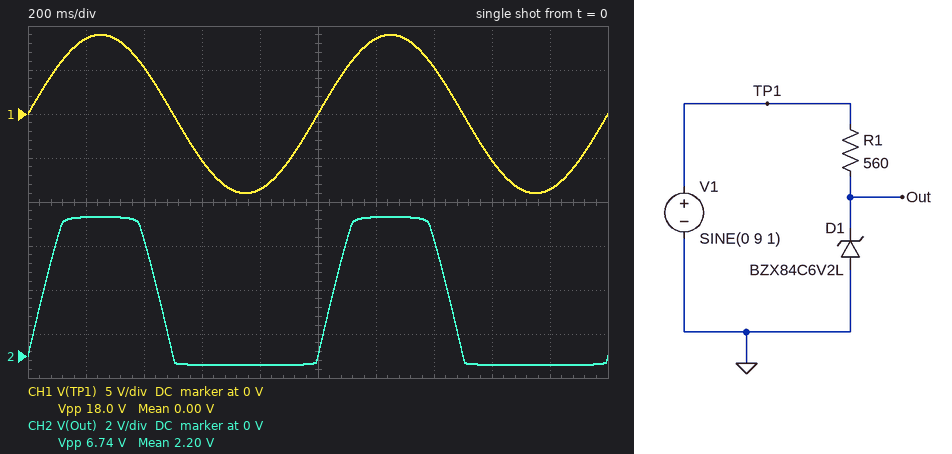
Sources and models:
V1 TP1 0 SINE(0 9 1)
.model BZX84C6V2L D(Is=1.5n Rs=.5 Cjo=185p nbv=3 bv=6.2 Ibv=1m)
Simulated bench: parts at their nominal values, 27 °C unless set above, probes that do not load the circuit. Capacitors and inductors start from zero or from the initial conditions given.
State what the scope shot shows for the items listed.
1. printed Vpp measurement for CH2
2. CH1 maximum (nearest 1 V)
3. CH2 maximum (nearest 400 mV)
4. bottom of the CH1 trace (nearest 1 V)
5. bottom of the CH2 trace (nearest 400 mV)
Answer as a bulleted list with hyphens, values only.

- 6.74 V
- 9 V
- 6.4 V
- -9 V
- -400 mV
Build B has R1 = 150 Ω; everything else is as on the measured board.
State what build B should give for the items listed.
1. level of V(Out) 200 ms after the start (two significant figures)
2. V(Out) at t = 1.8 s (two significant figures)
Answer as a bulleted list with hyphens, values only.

- 6.4 V
- -480 mV
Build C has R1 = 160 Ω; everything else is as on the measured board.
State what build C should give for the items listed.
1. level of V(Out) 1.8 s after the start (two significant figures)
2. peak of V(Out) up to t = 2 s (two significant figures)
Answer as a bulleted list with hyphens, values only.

- -470 mV
- 6.4 V
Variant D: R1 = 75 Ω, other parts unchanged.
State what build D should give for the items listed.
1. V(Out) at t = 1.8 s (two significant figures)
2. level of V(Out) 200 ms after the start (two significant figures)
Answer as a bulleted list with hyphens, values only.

- -520 mV
- 6.5 V
